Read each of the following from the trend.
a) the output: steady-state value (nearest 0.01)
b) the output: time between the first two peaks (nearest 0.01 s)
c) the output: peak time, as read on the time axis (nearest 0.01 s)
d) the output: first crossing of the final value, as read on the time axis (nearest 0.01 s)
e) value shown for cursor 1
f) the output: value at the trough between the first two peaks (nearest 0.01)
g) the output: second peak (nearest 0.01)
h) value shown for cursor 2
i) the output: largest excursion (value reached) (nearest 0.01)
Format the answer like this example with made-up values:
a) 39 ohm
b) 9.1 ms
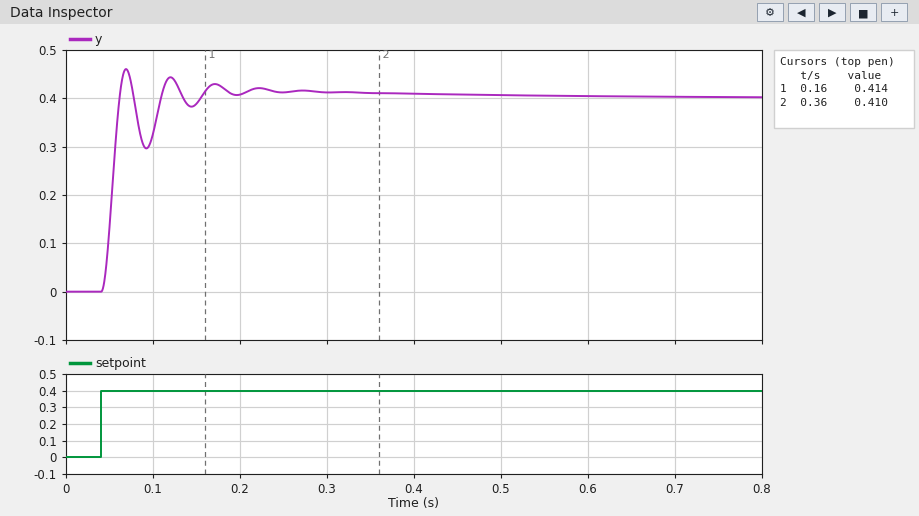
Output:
a) 0.40
b) 0.05 s
c) 0.07 s
d) 0.06 s
e) 0.414
f) 0.30
g) 0.44
h) 0.410
i) 0.46
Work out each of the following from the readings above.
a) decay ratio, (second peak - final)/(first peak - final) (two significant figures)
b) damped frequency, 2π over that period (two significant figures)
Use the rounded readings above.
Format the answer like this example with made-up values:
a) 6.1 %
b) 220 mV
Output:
a) 0.67
b) 130 rad/s
